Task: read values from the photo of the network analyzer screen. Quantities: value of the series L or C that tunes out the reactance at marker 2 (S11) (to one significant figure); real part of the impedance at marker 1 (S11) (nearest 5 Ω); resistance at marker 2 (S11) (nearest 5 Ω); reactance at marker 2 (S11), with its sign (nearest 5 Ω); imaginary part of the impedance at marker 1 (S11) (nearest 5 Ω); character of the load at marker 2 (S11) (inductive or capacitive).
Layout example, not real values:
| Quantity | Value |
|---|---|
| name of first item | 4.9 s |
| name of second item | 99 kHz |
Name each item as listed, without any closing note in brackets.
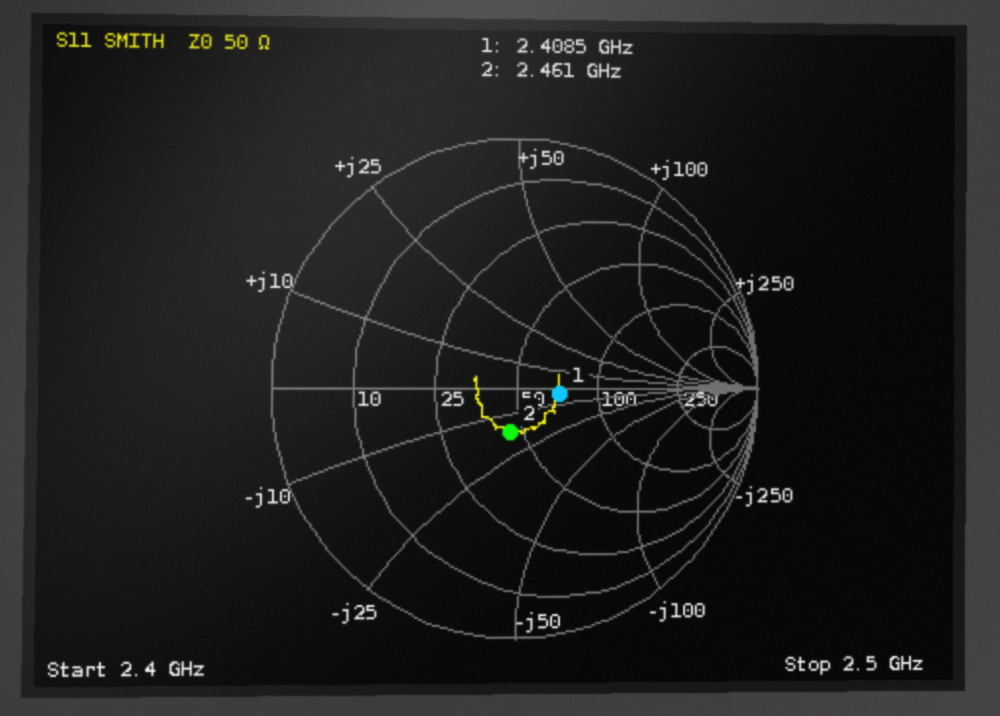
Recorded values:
| Quantity | Value |
|---|---|
| value of the series L or C that tunes out the reactance at marker 2 (S11) | 1 nH |
| real part of the impedance at marker 1 (S11) | 70 Ω |
| resistance at marker 2 (S11) | 45 Ω |
| reactance at marker 2 (S11), with its sign | -15 Ω |
| imaginary part of the impedance at marker 1 (S11) | -5 Ω |
| character of the load at marker 2 (S11) | capacitive |
